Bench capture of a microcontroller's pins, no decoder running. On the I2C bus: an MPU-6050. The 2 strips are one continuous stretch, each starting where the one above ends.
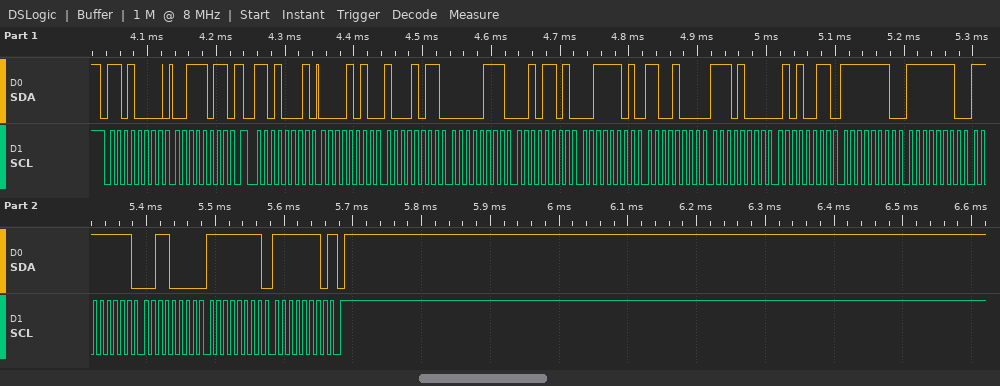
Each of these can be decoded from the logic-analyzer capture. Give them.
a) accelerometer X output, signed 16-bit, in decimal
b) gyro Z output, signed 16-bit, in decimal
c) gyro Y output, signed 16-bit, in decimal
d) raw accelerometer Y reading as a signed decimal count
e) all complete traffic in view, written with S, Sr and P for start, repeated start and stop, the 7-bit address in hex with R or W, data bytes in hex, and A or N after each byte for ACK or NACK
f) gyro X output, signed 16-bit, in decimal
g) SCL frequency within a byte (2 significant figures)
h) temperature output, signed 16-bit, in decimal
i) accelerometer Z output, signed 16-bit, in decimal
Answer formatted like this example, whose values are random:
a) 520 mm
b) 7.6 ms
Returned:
a) 2699
b) -2
c) -208
d) 1837
e) S 68W A 3B A Sr 68R A 0A A 8B A 07 A 2D A 3D A C8 A E8 A 53 A FE A FE A FF A 30 A FF A FE N P
f) -258
g) 100 kHz
h) -6061
i) 15816
